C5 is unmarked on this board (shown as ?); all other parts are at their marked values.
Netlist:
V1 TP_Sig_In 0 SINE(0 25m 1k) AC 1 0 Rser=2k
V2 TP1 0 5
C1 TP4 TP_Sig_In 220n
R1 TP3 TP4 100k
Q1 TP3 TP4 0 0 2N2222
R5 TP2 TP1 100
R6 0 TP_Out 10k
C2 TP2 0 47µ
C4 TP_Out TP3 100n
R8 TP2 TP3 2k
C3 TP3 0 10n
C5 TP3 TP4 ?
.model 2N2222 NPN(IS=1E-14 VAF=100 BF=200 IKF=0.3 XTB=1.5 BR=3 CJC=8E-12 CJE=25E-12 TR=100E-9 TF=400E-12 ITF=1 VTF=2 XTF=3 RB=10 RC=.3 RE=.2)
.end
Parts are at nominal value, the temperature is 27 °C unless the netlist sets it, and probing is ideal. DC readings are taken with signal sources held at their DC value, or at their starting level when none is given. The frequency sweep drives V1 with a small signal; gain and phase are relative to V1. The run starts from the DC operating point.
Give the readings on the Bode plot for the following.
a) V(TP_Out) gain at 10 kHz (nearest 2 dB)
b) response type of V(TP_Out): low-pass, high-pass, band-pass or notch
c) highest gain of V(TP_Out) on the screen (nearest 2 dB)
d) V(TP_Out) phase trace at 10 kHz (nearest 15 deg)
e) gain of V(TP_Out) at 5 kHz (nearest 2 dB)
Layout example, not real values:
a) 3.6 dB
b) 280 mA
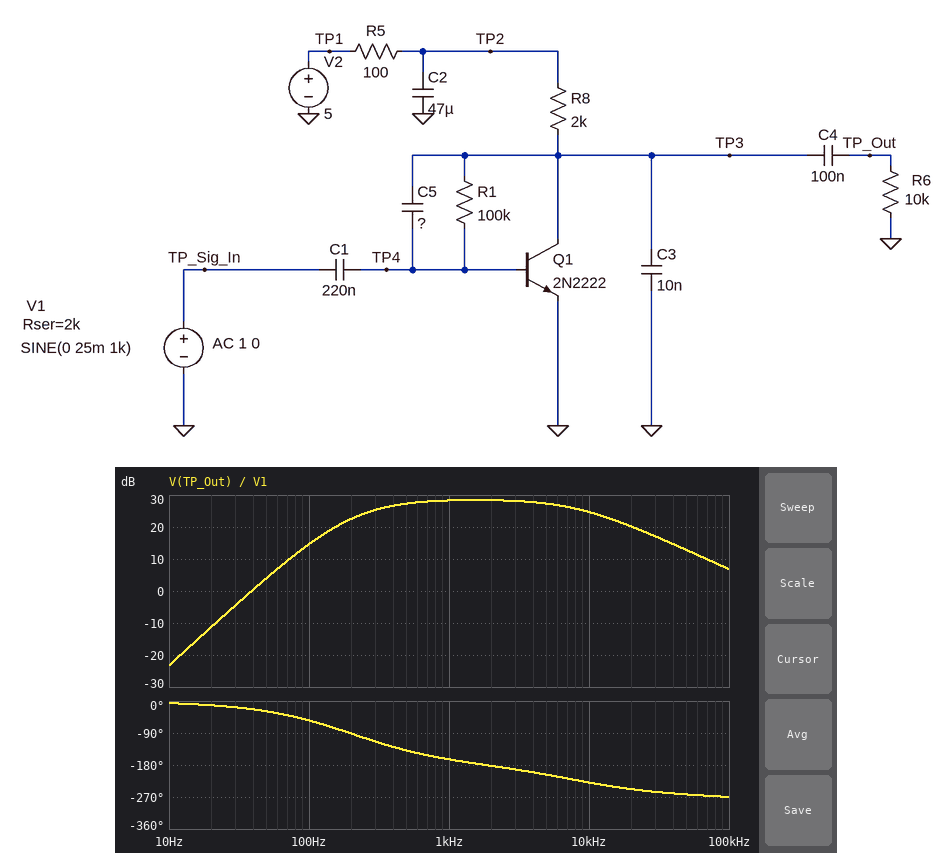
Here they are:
a) 24 dB
b) band-pass
c) 28 dB
d) -225 deg
e) 28 dB
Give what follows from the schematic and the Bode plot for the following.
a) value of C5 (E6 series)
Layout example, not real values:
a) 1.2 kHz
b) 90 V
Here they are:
a) 220 pF
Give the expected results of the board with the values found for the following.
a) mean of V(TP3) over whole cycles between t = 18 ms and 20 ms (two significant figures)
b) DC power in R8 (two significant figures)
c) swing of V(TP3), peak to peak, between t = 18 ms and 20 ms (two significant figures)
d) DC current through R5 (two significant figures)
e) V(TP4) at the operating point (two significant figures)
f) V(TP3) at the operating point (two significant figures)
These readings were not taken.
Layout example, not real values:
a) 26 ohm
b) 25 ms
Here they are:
a) 1.5 V
b) 5.6 mW
c) 1.3 V
d) 1.7 mA
e) 670 mV
f) 1.5 V
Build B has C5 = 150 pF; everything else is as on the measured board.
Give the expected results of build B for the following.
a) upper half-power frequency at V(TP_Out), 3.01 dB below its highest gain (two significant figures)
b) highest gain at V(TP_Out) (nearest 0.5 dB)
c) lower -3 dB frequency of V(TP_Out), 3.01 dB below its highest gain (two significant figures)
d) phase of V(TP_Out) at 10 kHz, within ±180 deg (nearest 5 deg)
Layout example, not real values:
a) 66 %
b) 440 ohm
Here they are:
a) 11 kHz
b) 28.5 dB
c) 310 Hz
d) 135 deg
